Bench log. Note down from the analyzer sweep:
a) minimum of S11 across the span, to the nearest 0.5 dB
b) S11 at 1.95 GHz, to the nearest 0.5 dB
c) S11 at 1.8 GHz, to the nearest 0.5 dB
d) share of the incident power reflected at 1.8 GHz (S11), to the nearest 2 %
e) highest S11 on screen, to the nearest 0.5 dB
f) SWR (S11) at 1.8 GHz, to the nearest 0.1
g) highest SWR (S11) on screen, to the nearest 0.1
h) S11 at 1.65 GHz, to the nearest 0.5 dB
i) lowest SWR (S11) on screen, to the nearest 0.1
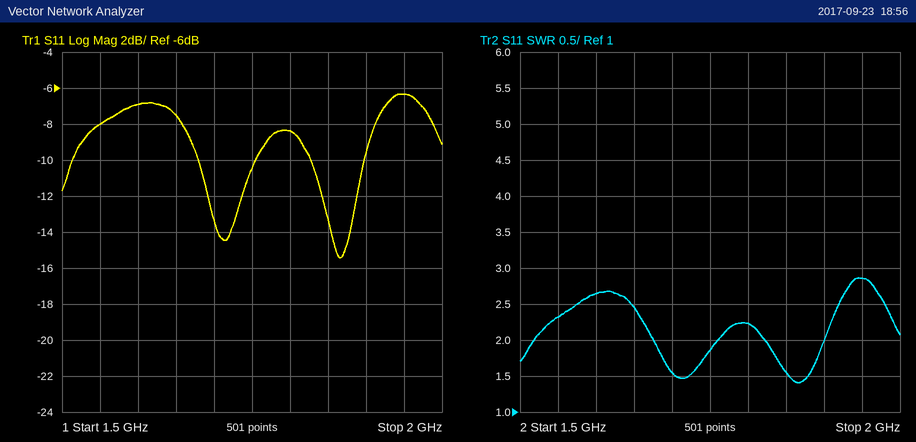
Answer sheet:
-15.5 dB
-6.5 dB
-8.5 dB
14 %
-6.5 dB
2.2
2.9
-7.5 dB
1.4
